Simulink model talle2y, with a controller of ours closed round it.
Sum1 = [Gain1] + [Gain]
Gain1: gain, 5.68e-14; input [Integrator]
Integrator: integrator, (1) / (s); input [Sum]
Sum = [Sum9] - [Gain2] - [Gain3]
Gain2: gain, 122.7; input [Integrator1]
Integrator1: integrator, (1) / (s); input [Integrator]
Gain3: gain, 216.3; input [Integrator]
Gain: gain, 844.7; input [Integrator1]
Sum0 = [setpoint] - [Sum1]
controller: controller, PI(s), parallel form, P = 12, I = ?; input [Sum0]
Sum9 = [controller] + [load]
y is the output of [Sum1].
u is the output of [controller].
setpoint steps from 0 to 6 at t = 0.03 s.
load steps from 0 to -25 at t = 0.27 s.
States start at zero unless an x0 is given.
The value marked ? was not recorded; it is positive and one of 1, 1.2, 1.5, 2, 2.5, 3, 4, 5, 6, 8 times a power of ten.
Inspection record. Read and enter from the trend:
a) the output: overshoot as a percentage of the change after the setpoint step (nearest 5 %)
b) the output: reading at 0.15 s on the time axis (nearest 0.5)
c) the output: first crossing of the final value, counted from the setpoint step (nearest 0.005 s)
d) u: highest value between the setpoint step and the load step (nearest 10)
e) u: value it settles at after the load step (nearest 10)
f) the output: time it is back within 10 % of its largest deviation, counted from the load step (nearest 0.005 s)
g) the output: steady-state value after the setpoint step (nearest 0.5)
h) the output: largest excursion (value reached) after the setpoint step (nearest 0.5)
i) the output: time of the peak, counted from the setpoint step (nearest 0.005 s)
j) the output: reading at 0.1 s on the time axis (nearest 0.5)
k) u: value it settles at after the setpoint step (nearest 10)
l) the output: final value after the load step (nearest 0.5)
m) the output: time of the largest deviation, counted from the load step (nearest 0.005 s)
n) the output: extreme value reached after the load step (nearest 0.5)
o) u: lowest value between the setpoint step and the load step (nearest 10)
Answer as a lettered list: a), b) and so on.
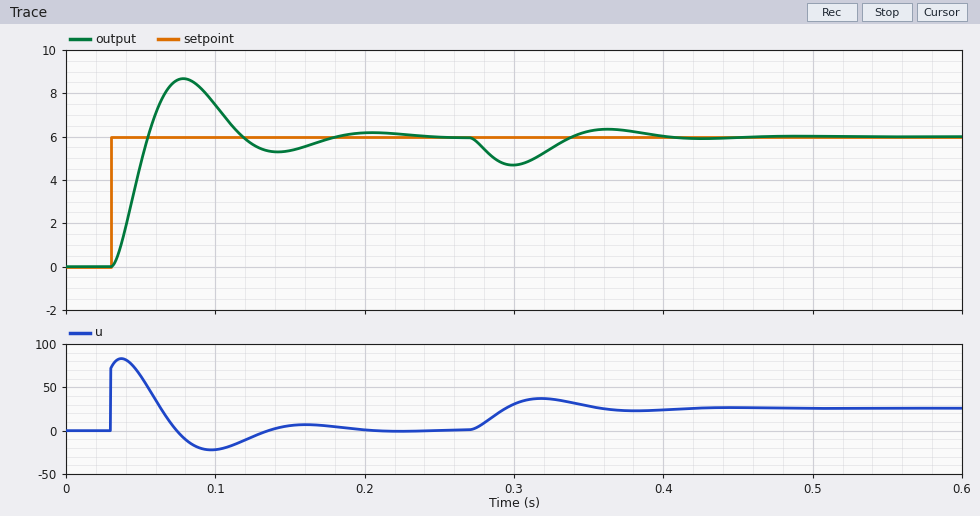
a) 45 %
b) 5.5
c) 0.025 s
d) 80
e) 30
f) 0.120 s
g) 6.0
h) 8.5
i) 0.050 s
j) 7.5
k) 0
l) 6.0
m) 0.030 s
n) 4.5
o) -20
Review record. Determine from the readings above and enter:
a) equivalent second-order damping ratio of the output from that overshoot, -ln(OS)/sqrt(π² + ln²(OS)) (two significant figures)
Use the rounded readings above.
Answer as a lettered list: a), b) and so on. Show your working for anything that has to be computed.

a) ln(0.45) = -0.799; 0.799 / sqrt(9.870 + 0.638) = 0.25
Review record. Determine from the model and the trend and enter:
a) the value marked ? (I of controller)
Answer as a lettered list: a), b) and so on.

a) 600
